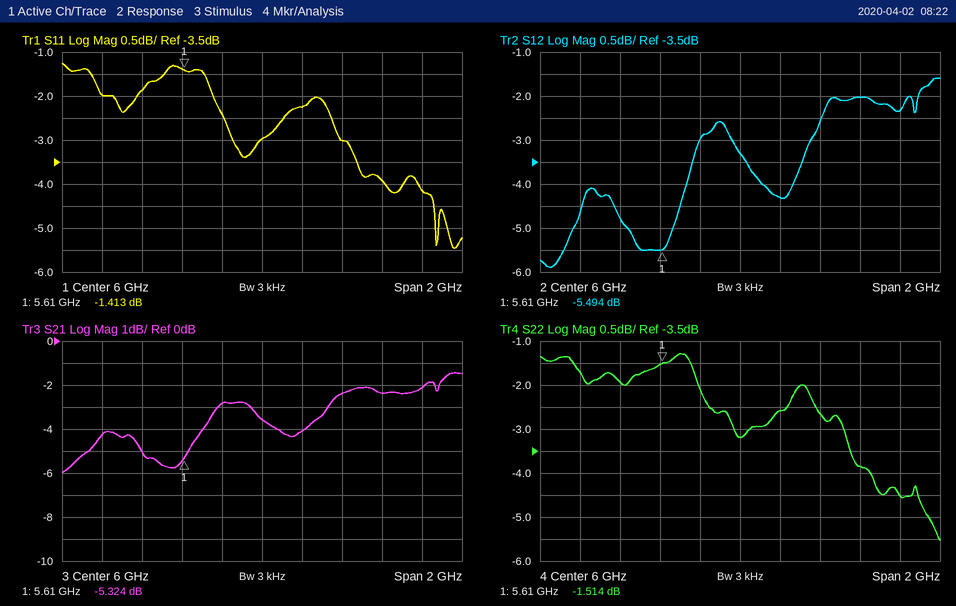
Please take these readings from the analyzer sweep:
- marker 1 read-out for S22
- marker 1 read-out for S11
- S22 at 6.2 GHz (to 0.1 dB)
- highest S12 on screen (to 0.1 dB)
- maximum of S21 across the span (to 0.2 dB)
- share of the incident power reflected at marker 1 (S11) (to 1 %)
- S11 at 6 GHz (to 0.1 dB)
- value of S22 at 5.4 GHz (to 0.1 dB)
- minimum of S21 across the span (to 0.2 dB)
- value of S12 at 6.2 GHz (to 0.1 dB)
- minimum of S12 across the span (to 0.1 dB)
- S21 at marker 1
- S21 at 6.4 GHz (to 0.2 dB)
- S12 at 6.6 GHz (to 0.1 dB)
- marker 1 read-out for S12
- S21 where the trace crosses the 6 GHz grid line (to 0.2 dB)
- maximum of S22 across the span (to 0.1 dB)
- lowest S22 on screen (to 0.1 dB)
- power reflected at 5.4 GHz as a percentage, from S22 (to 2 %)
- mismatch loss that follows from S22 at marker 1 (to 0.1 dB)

-1.514 dB
-1.413 dB
-2.6 dB
-1.6 dB
-1.4 dB
72 %
-3.0 dB
-1.9 dB
-6.0 dB
-4.3 dB
-5.9 dB
-5.324 dB
-2.4 dB
-2.0 dB
-5.494 dB
-3.6 dB
-1.3 dB
-5.5 dB
64 %
5.3 dB
